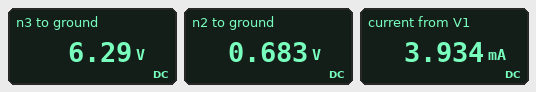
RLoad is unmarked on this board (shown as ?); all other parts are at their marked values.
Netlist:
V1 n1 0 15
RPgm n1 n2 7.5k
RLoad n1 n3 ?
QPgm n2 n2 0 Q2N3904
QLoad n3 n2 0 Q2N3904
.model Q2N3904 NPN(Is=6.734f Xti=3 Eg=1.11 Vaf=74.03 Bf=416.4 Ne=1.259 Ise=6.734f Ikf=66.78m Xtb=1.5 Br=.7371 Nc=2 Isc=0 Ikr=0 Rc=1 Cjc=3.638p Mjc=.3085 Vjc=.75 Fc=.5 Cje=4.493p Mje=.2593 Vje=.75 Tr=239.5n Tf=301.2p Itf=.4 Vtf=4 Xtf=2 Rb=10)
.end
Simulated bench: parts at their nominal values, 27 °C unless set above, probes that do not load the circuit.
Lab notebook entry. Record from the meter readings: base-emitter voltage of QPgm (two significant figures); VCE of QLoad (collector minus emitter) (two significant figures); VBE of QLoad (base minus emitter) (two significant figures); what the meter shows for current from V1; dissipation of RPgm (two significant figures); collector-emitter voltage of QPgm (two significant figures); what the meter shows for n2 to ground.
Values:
680 mV
6.3 V
680 mV
3.934 mA
27 mW
680 mV
0.683 V
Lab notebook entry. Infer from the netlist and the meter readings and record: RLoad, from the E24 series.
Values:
4.3 kΩ
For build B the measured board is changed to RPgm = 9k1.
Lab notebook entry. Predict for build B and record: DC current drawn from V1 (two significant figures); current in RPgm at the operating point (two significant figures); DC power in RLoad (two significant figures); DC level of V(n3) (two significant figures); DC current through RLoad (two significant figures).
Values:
3.3 mA
1.6 mA
12 mW
7.7 V
1.7 mA
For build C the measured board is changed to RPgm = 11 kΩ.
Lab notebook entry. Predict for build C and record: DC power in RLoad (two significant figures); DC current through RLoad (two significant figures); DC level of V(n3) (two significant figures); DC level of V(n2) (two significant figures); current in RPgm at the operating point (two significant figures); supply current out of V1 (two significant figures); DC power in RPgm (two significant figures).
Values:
8.7 mW
1.4 mA
8.9 V
670 mV
1.3 mA
2.7 mA
19 mW
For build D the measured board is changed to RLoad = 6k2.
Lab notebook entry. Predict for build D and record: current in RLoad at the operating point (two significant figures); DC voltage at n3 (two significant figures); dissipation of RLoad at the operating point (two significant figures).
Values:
1.9 mA
3.0 V
23 mW
